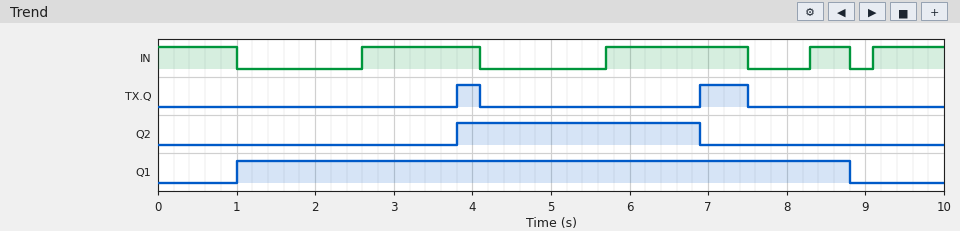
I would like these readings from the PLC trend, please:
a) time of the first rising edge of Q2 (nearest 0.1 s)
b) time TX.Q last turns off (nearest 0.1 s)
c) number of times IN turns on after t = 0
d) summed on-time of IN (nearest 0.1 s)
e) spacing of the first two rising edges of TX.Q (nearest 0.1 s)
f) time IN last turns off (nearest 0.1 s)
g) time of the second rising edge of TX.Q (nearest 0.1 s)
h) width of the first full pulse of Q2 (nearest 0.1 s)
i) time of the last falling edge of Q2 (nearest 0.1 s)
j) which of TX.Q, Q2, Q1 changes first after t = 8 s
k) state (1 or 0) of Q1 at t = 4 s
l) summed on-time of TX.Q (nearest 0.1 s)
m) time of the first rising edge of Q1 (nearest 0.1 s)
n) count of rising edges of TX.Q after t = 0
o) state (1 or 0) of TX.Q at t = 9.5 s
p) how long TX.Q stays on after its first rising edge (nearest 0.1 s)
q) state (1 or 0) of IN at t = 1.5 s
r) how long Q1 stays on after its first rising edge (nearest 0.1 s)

3.8 s
7.5 s
4
5.7 s
3.1 s
8.8 s
6.9 s
3.1 s
6.9 s
Q1
1
0.9 s
1.0 s
2
0
0.3 s
0
7.8 s
